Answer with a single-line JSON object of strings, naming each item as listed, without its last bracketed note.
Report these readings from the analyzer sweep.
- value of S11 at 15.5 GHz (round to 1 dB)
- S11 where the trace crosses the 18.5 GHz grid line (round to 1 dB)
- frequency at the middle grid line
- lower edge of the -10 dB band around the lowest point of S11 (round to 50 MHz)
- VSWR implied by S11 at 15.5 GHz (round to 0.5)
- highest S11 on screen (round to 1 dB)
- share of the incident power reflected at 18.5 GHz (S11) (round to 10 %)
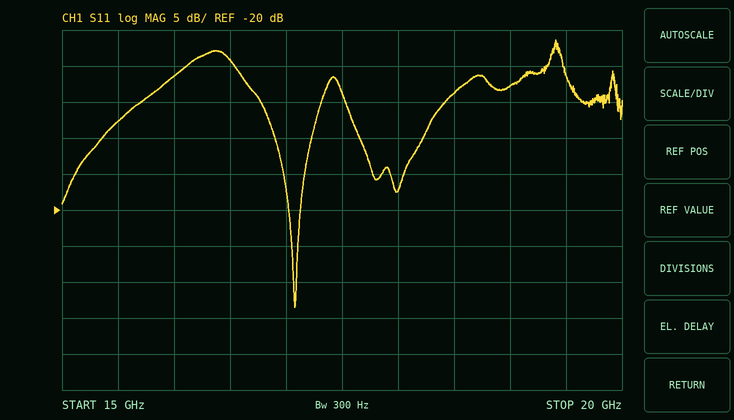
{"value of S11 at 15.5 GHz": "-8 dB", "S11 where the trace crosses the 18.5 GHz grid line": "-4 dB", "frequency at the middle grid line": "17.5 GHz", "lower edge of the -10 dB band around the lowest point of S11": "16.90 GHz", "VSWR implied by S11 at 15.5 GHz": "2.5", "highest S11 on screen": "4 dB", "share of the incident power reflected at 18.5 GHz (S11)": "40 %"}
